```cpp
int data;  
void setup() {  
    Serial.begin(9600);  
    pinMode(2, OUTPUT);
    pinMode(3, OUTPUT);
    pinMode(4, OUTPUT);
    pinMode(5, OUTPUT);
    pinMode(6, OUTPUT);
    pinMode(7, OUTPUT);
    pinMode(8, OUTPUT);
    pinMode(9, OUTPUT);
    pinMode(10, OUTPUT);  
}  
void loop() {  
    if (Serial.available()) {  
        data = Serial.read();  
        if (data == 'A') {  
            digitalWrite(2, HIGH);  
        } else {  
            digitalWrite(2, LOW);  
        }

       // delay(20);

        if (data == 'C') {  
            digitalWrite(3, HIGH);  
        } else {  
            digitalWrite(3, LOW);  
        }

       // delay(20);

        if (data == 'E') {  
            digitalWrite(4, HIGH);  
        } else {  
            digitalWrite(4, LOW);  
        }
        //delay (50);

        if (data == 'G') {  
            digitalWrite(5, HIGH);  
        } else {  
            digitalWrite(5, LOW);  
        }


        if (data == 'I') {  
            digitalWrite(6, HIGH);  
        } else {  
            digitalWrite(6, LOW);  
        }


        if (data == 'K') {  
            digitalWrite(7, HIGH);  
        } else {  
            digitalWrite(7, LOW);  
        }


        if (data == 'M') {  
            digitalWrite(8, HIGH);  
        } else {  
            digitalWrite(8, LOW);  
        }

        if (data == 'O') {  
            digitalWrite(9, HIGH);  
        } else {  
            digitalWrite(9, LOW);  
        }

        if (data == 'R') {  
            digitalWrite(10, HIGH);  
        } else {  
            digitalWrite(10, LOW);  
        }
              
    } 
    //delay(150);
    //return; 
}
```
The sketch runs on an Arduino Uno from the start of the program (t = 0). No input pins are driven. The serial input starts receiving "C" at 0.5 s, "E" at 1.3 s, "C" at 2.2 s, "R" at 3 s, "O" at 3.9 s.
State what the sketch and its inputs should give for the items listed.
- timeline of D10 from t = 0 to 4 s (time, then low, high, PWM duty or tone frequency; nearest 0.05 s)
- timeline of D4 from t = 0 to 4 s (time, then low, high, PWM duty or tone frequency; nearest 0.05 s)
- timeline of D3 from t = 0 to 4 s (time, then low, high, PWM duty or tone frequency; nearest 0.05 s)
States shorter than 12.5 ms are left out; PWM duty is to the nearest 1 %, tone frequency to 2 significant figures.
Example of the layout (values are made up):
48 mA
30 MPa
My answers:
0 s low; 3 s high; 3.9 s low
0 s low; 1.3 s high; 2.2 s low
0 s low; 0.5 s high; 1.3 s low; 2.2 s high; 3 s low
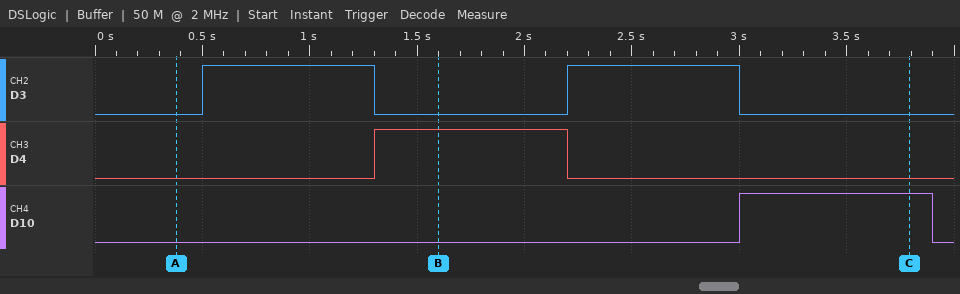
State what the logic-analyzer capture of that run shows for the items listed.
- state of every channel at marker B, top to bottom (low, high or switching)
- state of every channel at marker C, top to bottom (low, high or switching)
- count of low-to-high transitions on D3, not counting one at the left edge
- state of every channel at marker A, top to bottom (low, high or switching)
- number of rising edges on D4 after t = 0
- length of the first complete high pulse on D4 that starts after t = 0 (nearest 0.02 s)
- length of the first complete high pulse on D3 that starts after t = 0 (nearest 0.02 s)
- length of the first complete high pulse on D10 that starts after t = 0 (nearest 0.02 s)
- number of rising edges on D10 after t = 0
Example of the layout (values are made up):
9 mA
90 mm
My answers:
D3 low, D4 high, D10 low
D3 low, D4 low, D10 high
2
D3 low, D4 low, D10 low
1
0.90 s
0.80 s
0.90 s
1
